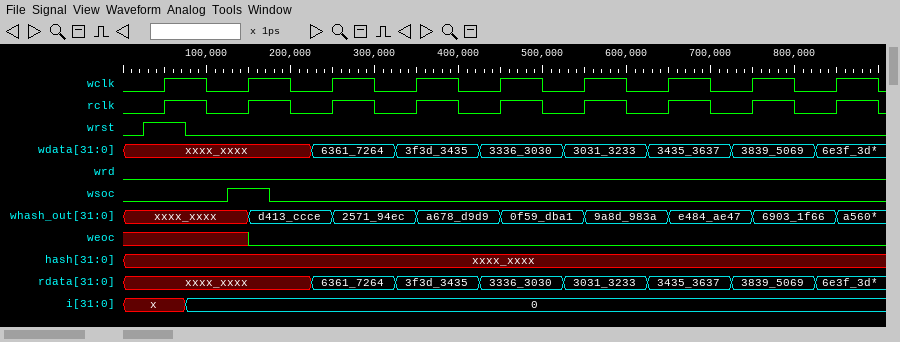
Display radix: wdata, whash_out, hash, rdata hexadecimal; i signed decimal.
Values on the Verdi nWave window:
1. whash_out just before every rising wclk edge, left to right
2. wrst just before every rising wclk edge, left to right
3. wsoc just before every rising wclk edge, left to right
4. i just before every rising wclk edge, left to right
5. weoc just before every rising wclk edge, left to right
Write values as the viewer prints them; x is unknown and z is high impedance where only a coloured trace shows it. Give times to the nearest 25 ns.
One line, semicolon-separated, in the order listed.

xxxx_xxxx, xxxx_xxxx, d413_ccce, 2571_94ec, a678_d9d9, 0f59_dba1, 9a8d_983a, e484_ae47, 6903_1f66; 1 0 0 0 0 0 0 0 0; 0 1 0 0 0 0 0 0 0; x, 0, 0, 0, 0, 0, 0, 0, 0; x x 0 0 0 0 0 0 0
